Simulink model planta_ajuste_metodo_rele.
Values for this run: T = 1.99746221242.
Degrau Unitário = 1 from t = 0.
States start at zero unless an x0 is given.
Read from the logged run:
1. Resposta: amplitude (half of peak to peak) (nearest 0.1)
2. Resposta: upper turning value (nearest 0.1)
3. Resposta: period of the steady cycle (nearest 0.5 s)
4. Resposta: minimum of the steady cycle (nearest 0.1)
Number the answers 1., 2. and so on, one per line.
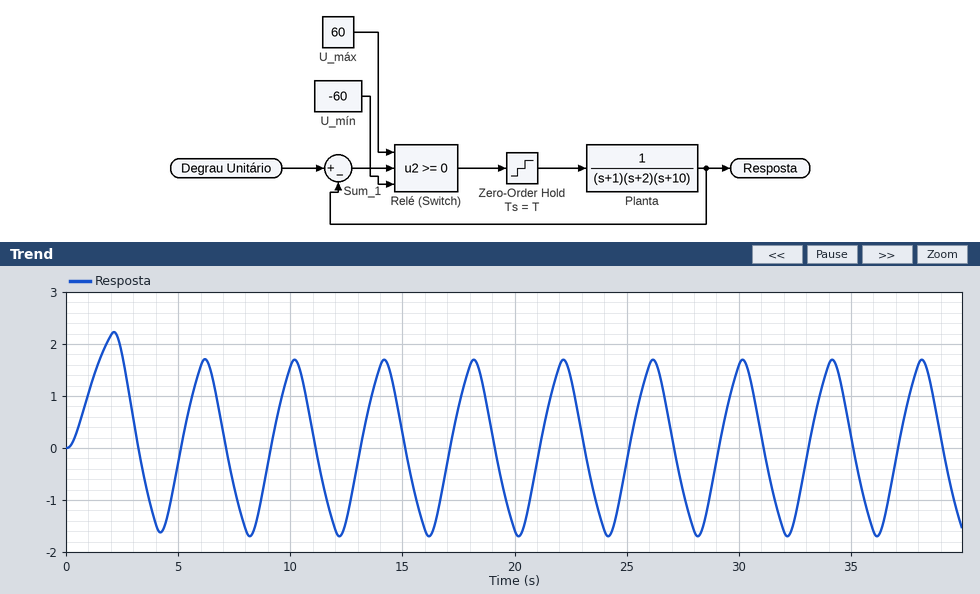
1. 1.7
2. 1.7
3. 4.0 s
4. -1.7
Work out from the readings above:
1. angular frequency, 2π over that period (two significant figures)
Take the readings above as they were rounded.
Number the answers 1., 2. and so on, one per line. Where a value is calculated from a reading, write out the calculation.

1. 2π / 4 = 1.6 rad/s
